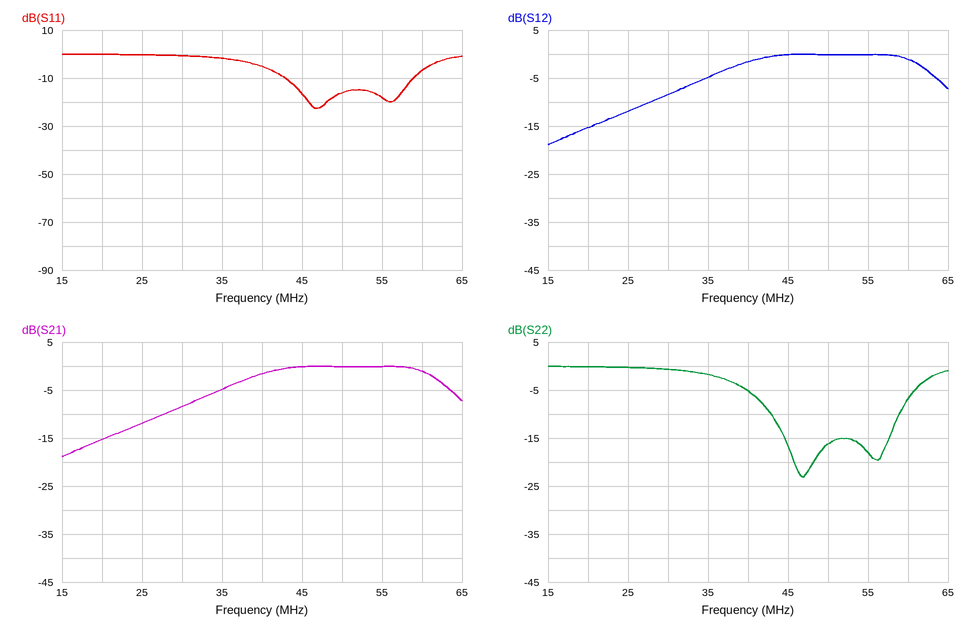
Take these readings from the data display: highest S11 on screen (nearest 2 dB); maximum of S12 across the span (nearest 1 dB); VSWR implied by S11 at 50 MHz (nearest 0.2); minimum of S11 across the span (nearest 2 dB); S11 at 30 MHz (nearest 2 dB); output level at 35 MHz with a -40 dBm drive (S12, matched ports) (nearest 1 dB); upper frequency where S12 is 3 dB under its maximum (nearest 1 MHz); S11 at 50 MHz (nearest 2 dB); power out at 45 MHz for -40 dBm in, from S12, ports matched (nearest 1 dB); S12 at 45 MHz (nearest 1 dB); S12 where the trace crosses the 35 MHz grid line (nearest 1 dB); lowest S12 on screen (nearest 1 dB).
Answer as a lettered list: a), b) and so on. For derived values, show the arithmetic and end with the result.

a) 0 dB
b) 0 dB
c) |Γ| = 10^(-16/20) = 0.1585; VSWR = (1 + 0.1585)/(1 − 0.1585) ≈ 1.4
d) -22 dB
e) 0 dB
f) -40 dBm + (-5 dB) = -45 dBm
g) 62 MHz
h) -16 dB
i) -40 dBm + (0 dB) = -40 dBm
j) 0 dB
k) -5 dB
l) -19 dB
